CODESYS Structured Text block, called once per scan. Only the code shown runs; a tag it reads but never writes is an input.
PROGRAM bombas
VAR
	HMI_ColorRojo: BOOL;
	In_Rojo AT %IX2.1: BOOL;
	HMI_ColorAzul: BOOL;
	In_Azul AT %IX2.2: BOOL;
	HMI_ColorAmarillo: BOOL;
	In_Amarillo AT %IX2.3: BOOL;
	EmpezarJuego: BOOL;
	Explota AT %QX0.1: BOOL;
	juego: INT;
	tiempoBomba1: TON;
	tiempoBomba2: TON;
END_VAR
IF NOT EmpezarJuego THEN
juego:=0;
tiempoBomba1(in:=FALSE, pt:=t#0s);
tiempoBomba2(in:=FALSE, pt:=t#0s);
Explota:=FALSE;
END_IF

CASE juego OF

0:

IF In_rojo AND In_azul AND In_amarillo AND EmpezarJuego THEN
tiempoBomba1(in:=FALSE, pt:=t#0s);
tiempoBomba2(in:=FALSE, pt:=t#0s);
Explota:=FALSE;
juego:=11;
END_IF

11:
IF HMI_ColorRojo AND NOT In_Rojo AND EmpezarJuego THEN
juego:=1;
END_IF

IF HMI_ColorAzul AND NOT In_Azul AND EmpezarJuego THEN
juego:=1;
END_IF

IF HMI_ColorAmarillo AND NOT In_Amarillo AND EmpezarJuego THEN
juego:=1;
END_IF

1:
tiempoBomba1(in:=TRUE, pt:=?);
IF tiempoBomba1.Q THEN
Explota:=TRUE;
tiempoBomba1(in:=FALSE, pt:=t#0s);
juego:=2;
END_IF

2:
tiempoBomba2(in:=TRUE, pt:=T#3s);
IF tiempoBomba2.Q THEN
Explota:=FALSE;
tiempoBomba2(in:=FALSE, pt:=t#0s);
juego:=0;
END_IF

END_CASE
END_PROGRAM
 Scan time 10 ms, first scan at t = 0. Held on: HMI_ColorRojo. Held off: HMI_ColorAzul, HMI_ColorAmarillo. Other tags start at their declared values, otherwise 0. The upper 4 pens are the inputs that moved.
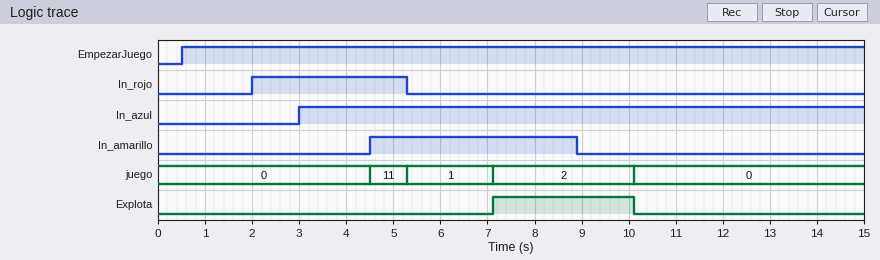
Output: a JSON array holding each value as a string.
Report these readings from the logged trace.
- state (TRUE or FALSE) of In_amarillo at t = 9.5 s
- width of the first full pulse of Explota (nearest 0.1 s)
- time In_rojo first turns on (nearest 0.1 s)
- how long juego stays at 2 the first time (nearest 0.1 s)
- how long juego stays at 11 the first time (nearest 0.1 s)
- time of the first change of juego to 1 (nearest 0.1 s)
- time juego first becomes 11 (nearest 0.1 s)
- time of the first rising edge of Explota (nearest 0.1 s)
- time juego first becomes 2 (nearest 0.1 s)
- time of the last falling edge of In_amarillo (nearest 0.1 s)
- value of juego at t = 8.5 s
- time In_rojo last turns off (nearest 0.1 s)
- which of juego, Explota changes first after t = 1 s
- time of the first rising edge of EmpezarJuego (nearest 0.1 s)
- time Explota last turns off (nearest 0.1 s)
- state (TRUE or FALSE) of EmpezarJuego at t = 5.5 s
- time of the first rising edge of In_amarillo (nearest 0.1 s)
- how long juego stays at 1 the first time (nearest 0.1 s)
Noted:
["FALSE", "3.0 s", "2.0 s", "3.0 s", "0.8 s", "5.3 s", "4.5 s", "7.1 s", "7.1 s", "8.9 s", "2", "5.3 s", "juego", "0.5 s", "10.1 s", "TRUE", "4.5 s", "1.8 s"]
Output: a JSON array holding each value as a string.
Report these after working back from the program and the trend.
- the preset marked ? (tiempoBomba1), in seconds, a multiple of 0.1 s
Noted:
["1.8 s"]
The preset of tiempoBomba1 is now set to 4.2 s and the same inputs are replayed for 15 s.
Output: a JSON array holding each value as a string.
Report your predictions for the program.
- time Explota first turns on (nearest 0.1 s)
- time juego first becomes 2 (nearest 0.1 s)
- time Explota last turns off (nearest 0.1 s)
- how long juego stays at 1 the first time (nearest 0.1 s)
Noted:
["9.5 s", "9.5 s", "12.5 s", "4.2 s"]
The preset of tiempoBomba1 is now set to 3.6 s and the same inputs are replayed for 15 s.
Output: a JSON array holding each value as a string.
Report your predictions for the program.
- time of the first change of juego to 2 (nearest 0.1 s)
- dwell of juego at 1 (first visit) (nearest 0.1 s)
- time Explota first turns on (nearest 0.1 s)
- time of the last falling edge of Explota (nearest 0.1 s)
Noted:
["8.9 s", "3.6 s", "8.9 s", "11.9 s"]
